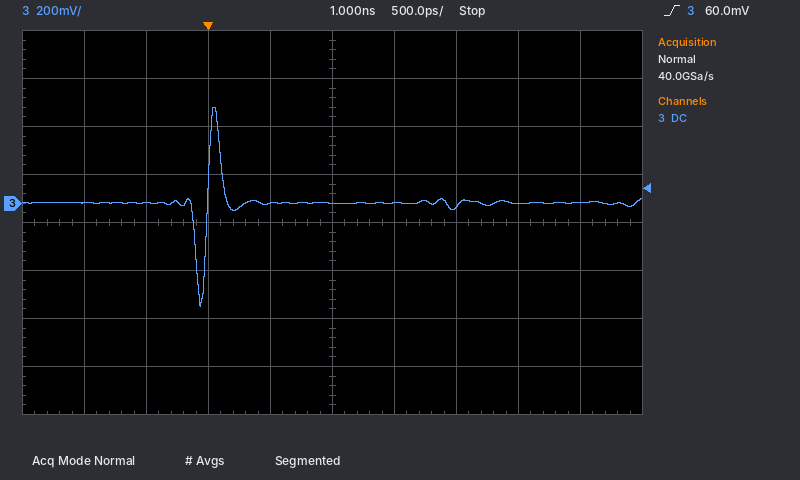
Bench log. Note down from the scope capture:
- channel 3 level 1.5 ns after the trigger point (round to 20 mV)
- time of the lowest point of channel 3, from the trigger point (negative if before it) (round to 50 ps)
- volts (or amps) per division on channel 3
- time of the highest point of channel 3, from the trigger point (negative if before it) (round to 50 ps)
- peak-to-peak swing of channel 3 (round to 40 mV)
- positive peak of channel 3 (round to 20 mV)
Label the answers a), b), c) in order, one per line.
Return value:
a) 0 mV
b) -50 ps
c) 200 mV
d) +50 ps
e) 840 mV
f) 400 mV
